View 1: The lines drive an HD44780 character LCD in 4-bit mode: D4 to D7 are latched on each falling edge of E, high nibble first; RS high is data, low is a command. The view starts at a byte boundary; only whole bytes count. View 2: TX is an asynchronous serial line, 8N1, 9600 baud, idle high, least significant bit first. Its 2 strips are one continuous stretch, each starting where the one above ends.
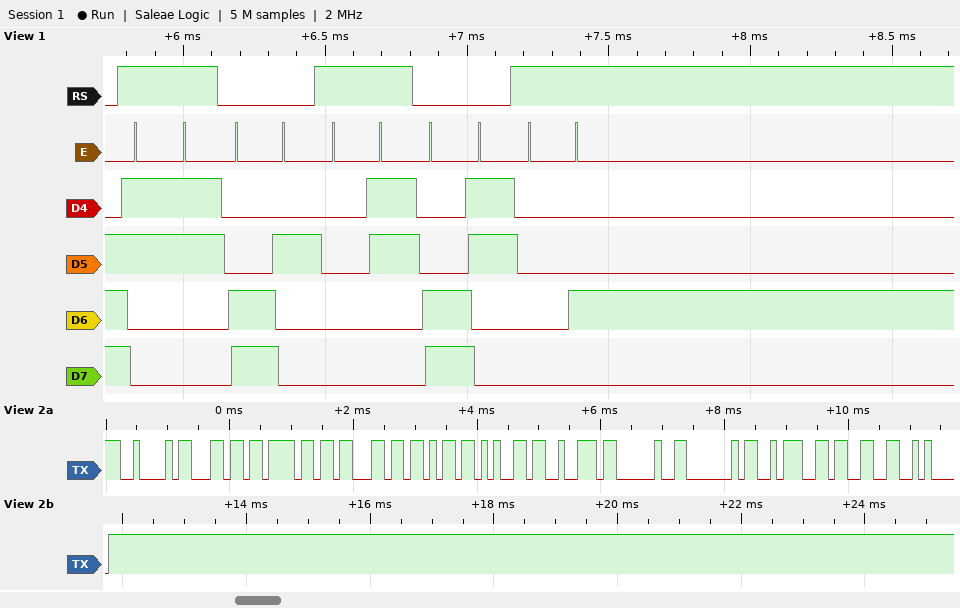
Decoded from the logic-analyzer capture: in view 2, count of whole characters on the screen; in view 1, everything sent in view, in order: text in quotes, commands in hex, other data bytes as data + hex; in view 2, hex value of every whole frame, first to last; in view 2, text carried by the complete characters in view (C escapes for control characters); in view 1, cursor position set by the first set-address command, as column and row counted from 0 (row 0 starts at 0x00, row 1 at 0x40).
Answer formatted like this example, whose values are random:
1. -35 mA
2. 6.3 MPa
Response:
1. 12
2. "3" 0xC2 data 03 0xC3 data 04
3. 0x42 0x6C 0x6F 0x63 0x6B 0x65 0x72 0x20 0x40 0x3A 0x33 0x0A
4. "Blocker @:3\n"
5. column 2, row 1
